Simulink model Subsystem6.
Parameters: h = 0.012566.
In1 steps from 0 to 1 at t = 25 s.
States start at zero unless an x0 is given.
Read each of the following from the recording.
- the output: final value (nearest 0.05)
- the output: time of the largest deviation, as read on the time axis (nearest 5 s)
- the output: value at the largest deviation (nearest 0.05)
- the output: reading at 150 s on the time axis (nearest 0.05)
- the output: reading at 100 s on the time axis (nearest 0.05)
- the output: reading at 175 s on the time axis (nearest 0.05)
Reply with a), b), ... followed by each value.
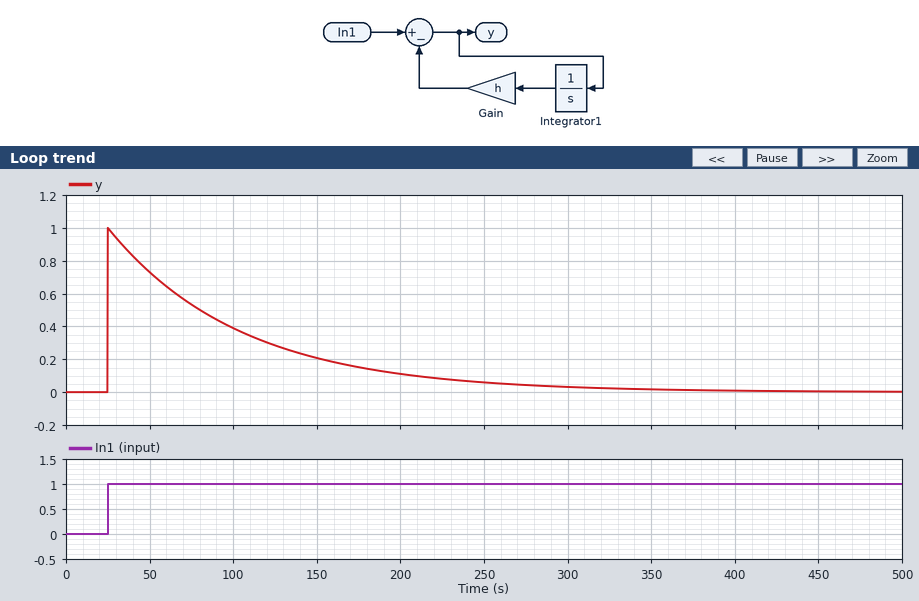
a) 0.00
b) 25 s
c) 1.00
d) 0.20
e) 0.40
f) 0.15
